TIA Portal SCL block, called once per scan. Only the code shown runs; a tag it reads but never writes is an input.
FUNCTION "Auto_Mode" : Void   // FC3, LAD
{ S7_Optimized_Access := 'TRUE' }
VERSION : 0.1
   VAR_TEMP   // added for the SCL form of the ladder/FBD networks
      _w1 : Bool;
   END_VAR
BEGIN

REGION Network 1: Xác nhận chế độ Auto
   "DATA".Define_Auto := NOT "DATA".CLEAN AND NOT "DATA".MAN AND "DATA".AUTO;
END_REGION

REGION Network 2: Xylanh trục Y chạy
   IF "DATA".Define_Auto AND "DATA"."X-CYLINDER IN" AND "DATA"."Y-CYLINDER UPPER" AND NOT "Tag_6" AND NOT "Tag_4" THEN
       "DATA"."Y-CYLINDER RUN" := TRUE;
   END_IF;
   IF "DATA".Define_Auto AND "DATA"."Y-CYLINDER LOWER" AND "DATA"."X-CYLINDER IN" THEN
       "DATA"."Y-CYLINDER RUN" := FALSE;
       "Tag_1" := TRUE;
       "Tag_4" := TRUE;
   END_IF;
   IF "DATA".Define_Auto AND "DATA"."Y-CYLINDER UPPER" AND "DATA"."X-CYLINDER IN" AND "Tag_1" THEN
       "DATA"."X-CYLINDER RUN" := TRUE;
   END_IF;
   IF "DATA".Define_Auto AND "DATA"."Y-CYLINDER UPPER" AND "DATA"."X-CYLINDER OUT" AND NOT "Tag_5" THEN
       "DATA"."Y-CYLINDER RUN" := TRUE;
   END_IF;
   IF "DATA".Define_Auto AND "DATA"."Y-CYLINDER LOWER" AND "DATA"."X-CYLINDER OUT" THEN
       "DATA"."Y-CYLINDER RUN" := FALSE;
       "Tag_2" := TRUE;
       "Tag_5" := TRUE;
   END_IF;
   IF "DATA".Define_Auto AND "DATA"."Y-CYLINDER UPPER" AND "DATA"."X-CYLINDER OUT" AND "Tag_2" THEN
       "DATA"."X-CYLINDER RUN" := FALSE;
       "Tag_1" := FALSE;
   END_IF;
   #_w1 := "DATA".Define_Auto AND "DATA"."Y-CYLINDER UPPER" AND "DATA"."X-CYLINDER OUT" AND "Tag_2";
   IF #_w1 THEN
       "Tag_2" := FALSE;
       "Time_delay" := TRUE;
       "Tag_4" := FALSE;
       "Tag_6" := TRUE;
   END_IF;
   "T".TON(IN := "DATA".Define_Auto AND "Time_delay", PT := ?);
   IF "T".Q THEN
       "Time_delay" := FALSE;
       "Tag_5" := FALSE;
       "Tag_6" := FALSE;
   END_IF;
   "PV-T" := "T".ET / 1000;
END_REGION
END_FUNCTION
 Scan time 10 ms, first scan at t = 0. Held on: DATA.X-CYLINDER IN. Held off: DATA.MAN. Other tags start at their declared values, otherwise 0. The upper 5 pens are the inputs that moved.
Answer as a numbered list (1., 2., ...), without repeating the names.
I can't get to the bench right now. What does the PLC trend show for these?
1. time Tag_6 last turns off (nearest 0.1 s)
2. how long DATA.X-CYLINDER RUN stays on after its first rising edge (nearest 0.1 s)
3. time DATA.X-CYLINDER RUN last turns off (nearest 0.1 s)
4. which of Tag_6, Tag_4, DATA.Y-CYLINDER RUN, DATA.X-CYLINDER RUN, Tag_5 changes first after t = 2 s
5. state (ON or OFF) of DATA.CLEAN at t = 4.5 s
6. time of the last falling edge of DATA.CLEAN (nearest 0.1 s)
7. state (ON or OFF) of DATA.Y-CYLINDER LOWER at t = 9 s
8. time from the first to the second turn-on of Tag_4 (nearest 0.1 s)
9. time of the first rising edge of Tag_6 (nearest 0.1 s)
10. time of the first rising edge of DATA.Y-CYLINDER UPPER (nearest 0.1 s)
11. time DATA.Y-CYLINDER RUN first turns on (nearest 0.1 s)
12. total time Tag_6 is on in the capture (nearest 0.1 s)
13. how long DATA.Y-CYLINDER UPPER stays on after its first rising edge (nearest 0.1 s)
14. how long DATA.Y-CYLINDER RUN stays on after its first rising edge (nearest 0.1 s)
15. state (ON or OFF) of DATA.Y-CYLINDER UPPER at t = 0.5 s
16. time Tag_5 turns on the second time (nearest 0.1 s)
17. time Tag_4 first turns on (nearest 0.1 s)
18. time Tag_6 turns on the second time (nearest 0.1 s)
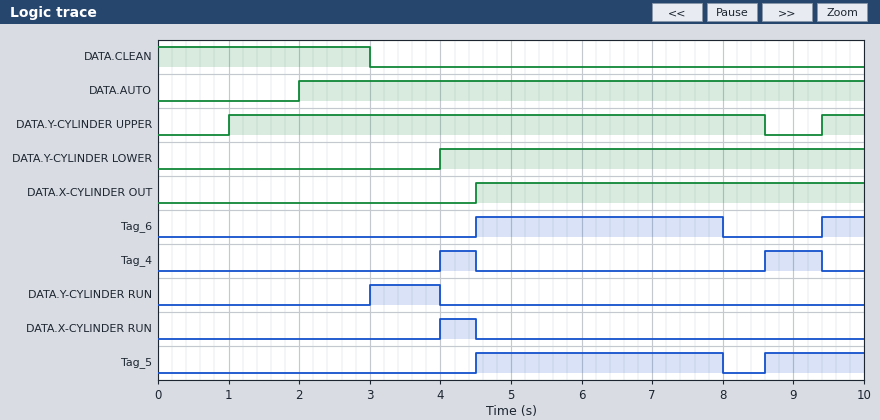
1. 8.0 s
2. 0.5 s
3. 4.5 s
4. DATA.Y-CYLINDER RUN
5. OFF
6. 3.0 s
7. ON
8. 4.6 s
9. 4.5 s
10. 1.0 s
11. 3.0 s
12. 4.1 s
13. 7.6 s
14. 1.0 s
15. OFF
16. 8.6 s
17. 4.0 s
18. 9.4 s
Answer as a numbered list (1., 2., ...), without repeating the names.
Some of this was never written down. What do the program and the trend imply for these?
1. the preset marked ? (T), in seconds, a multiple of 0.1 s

1. 3.5 s
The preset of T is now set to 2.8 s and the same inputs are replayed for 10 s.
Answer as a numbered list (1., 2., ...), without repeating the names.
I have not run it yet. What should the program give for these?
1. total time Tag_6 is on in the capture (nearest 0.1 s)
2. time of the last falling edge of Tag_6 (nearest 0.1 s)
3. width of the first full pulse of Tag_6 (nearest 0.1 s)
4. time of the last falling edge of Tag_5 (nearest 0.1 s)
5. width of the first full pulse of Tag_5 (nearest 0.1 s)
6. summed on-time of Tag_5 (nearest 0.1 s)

1. 3.4 s
2. 7.3 s
3. 2.8 s
4. 7.3 s
5. 2.8 s
6. 4.2 s
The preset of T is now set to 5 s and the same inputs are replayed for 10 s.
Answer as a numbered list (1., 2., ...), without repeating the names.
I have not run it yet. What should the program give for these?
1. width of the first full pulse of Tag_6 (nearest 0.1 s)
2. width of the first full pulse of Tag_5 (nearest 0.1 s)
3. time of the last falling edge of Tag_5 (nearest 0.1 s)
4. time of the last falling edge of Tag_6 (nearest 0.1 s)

1. 5.0 s
2. 5.0 s
3. 9.5 s
4. 9.5 s
